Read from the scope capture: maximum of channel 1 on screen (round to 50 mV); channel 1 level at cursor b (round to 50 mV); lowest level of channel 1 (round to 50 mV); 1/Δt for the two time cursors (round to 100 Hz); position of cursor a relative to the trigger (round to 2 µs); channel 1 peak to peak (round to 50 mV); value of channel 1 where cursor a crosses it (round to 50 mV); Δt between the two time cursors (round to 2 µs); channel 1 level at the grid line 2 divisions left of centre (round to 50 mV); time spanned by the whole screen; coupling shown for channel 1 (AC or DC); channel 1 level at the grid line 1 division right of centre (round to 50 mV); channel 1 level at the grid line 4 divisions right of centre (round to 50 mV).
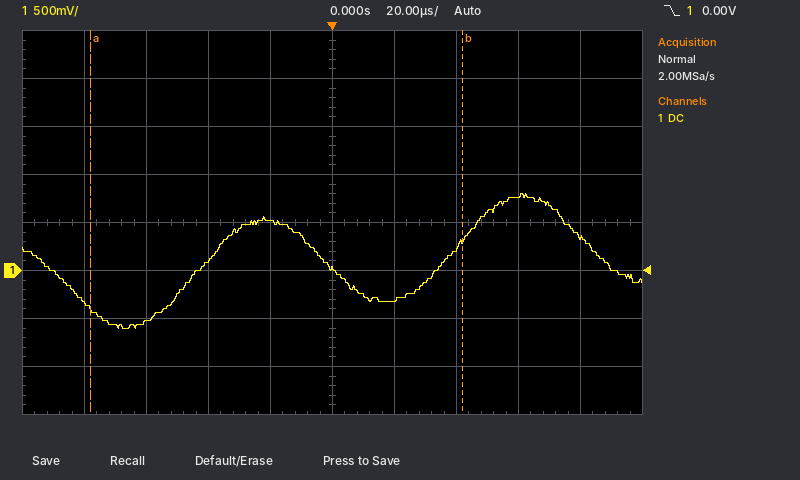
800 mV
300 mV
-600 mV
8.3 kHz
-78 µs
1.40 V
-400 mV
120 µs
100 mV
200 µs
DC
-300 mV
350 mV
